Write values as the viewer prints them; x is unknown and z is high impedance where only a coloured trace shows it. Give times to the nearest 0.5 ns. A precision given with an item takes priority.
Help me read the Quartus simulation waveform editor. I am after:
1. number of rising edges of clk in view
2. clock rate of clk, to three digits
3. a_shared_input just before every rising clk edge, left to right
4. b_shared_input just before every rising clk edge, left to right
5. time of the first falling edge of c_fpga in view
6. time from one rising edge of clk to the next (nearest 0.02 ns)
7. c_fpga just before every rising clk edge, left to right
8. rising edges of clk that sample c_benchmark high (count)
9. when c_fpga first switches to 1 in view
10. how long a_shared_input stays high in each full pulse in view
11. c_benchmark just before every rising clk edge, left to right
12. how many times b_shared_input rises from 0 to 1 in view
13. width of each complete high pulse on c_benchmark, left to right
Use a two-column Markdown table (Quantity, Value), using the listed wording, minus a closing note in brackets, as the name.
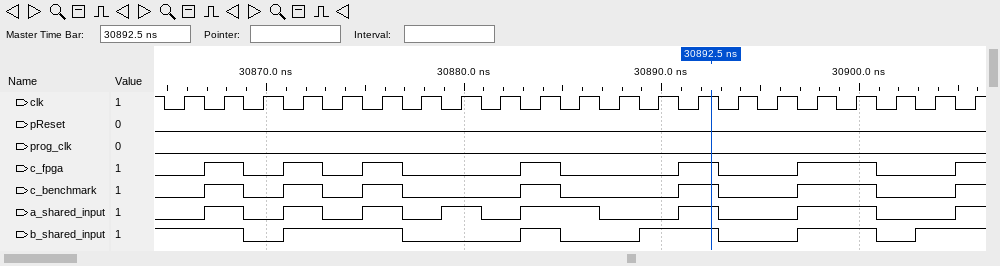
| Quantity | Value |
|---|---|
| number of rising edges of clk in view | 21 |
| clock rate of clk, to three digits | 500 MHz |
| a_shared_input just before every rising clk edge, left to right | 0 1 0 1 0 1 0 1 0 1 1 0 0 1 0 0 1 1 0 0 1 |
| b_shared_input just before every rising clk edge, left to right | 1 1 0 1 1 1 0 0 0 1 0 0 1 1 0 0 1 1 0 1 1 |
| time of the first falling edge of c_fpga in view | 30869 ns |
| time from one rising edge of clk to the next | 2 ns |
| c_fpga just before every rising clk edge, left to right | 0 1 0 1 0 1 0 0 0 1 0 0 0 1 0 0 1 1 0 0 1 |
| rising edges of clk that sample c_benchmark high | 8 |
| when c_fpga first switches to 1 in view | 30867 ns |
| how long a_shared_input stays high in each full pulse in view | 2 ns, 2 ns, 2 ns, 2 ns, 4 ns, 2 ns, 4 ns |
| c_benchmark just before every rising clk edge, left to right | 0 1 0 1 0 1 0 0 0 1 0 0 0 1 0 0 1 1 0 0 1 |
| how many times b_shared_input rises from 0 to 1 in view | 5 |
| width of each complete high pulse on c_benchmark, left to right | 2 ns, 2 ns, 2 ns, 2 ns, 2 ns, 4 ns |
